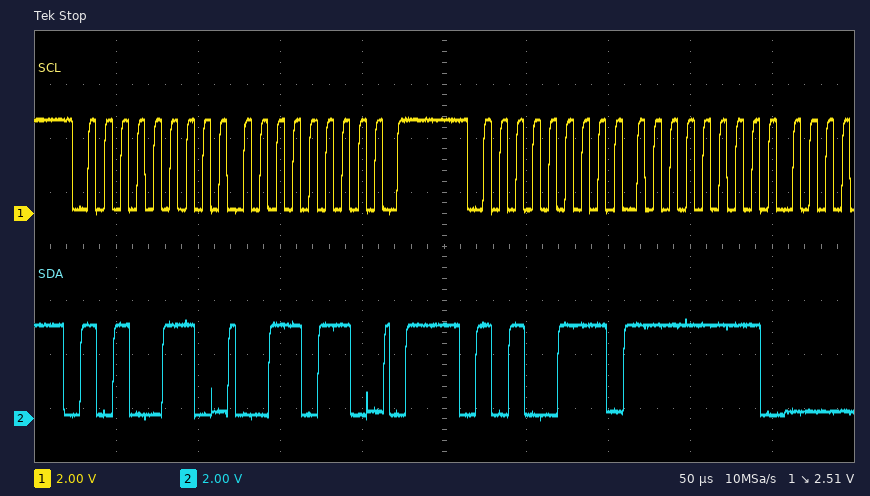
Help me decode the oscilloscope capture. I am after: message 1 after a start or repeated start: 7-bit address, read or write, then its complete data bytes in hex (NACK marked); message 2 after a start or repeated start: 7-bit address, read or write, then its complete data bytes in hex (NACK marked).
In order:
0x53 write: 36
0x53 read: FF
